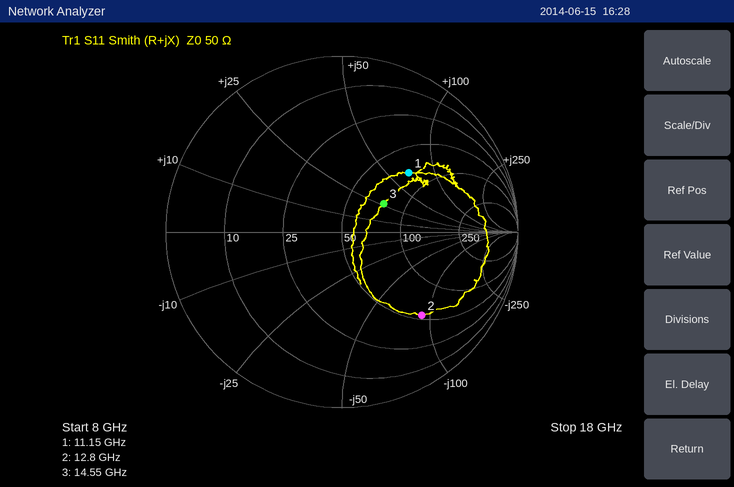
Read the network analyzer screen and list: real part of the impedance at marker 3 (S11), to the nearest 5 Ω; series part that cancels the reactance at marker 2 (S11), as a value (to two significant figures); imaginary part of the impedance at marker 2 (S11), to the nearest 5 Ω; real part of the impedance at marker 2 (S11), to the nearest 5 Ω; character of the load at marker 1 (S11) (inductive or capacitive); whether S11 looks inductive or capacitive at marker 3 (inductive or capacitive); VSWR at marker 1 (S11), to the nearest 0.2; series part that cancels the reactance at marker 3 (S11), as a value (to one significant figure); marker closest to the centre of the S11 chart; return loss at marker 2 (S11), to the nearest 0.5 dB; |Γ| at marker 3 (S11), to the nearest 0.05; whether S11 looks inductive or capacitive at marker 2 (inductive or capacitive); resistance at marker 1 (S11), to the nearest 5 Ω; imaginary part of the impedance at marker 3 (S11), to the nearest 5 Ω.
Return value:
75 Ω
1.1 nH
-90 Ω
55 Ω
inductive
inductive
3.0
400 fF
marker 3
3.5 dB
0.30
capacitive
75 Ω
+25 Ω
